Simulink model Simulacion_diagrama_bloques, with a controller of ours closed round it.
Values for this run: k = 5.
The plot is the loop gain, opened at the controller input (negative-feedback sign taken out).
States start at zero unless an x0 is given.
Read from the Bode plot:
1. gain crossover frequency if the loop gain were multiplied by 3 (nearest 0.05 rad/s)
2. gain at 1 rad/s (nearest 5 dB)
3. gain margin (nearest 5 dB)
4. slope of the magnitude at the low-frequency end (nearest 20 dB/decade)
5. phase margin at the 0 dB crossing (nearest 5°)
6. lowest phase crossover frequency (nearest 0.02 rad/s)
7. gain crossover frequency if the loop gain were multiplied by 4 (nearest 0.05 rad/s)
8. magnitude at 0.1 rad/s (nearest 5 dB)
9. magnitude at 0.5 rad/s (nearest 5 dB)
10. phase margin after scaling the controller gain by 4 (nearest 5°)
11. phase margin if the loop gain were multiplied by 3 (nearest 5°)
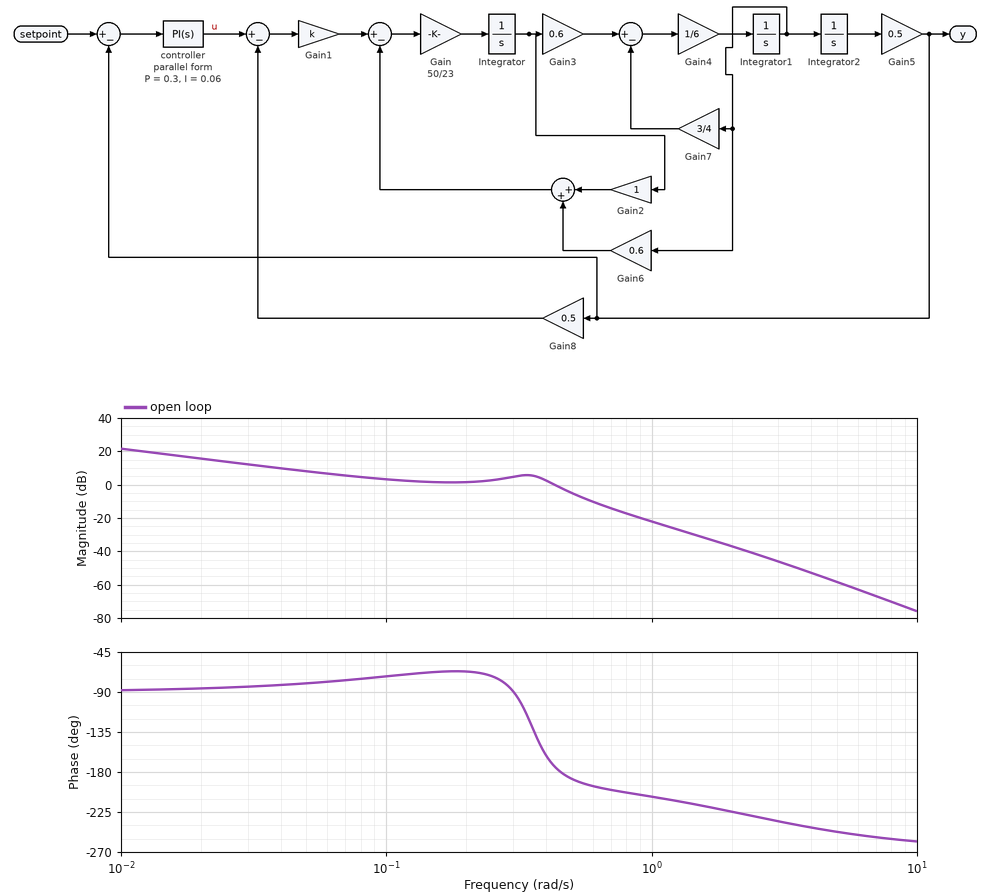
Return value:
0.60 rad/s
-20 dB
0 dB
-20 dB/decade
5°
0.46 rad/s
0.65 rad/s
5 dB
-5 dB
-20°
-15°
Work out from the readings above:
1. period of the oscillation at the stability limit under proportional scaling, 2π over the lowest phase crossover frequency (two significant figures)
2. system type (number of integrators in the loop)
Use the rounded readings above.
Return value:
14 s
1
